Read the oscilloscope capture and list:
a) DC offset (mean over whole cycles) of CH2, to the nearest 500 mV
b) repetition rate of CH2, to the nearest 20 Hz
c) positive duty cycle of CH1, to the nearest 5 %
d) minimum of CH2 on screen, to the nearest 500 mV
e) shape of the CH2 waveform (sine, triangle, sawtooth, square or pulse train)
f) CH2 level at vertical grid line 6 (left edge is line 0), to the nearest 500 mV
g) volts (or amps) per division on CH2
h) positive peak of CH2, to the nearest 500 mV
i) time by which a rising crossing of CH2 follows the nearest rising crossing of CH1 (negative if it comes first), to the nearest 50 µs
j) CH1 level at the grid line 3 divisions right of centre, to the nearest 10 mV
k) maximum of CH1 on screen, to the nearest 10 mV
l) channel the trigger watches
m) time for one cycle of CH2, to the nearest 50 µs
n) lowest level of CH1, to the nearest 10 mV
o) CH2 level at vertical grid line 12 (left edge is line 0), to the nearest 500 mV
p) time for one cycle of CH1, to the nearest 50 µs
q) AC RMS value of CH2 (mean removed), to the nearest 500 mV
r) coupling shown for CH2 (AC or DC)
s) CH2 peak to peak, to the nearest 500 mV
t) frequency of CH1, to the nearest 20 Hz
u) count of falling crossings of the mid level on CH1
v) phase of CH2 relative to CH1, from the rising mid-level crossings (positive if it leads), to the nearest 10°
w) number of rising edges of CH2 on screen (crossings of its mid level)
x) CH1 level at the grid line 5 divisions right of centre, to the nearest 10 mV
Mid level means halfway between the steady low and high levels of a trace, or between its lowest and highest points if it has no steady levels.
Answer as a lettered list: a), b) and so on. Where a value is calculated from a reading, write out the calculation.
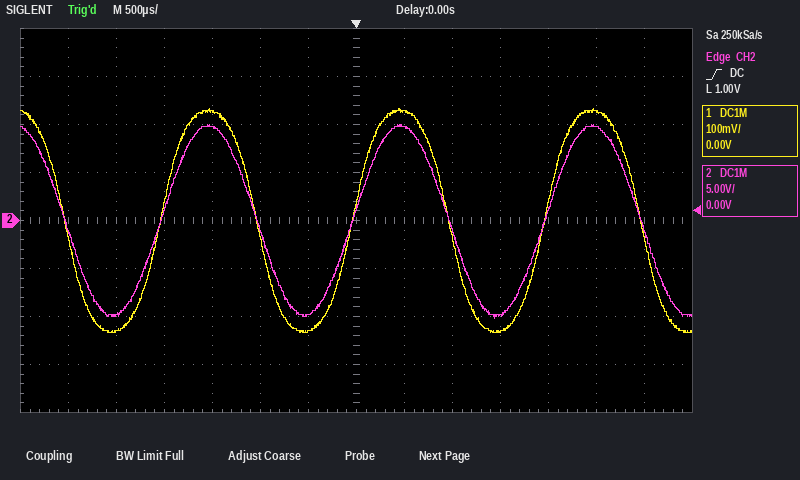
a) (10.0 V + (-10.0 V)) / 2 ≈ 0.0 V
b) 1 / 2.00 ms ≈ 500 Hz
c) 50 %
d) -10.0 V
e) sine
f) -10.0 V
g) 5 V
h) 10.0 V
i) 0 µs
j) -230 mV
k) 230 mV
l) CH2
m) 2.00 ms
n) -230 mV
o) 10.0 V
p) 2.00 ms
q) 20.0 V / (2√2) ≈ 7.07 V, so 7.0 V to the nearest 500 mV
r) DC
s) 10.0 V − (-10.0 V) = 20.0 V
t) 1 / 2.00 ms ≈ 500 Hz
u) 4
v) −360° × (0 µs) / 2.00 ms ≈ 0°
w) 3
x) 230 mV
